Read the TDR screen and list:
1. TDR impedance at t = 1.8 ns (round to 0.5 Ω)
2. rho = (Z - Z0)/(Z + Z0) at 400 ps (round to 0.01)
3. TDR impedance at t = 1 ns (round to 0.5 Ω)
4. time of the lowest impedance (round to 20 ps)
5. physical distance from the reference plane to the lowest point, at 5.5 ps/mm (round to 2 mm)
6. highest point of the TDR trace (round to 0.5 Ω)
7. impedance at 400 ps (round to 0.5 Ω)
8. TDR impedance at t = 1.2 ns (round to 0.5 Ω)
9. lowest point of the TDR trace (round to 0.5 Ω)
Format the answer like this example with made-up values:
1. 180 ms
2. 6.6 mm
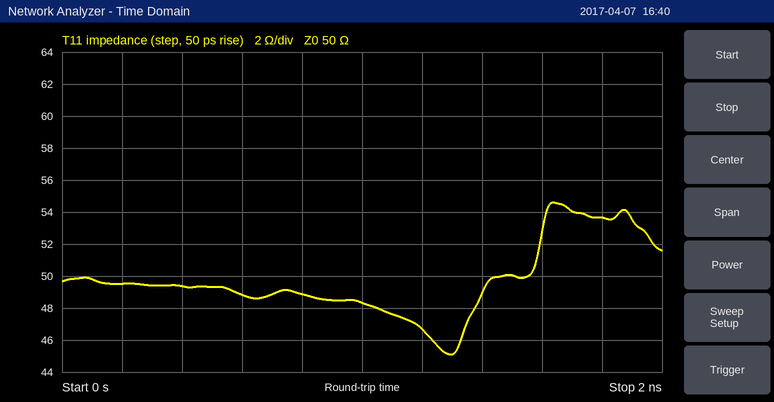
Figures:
1. 53.5 Ω
2. -0.01
3. 48.5 Ω
4. 1.30 ns
5. 118 mm
6. 54.5 Ω
7. 49.5 Ω
8. 46.5 Ω
9. 45.0 Ω
